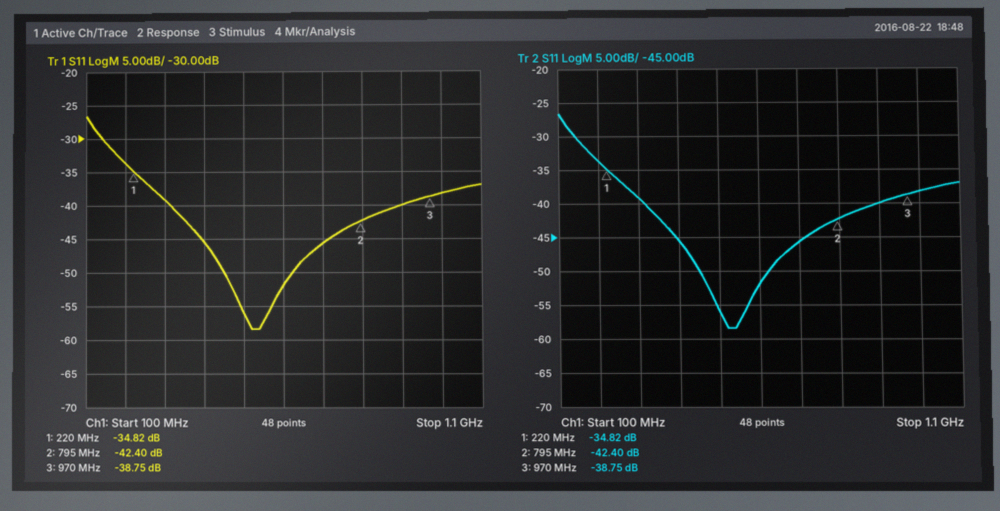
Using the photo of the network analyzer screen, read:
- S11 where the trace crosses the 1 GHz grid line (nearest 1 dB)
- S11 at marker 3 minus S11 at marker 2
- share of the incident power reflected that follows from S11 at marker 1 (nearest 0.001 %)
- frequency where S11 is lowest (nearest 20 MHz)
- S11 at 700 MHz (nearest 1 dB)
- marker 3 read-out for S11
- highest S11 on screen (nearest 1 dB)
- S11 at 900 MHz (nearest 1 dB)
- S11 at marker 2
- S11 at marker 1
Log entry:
-38 dB
3.65 dB
0.033 %
520 MHz
-46 dB
-38.75 dB
-27 dB
-40 dB
-42.40 dB
-34.82 dB
